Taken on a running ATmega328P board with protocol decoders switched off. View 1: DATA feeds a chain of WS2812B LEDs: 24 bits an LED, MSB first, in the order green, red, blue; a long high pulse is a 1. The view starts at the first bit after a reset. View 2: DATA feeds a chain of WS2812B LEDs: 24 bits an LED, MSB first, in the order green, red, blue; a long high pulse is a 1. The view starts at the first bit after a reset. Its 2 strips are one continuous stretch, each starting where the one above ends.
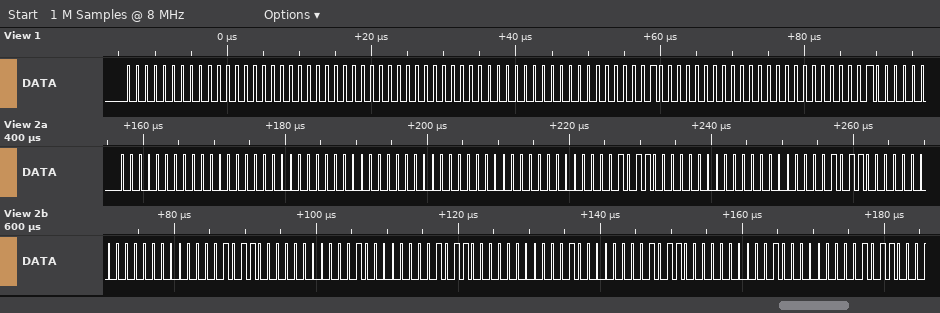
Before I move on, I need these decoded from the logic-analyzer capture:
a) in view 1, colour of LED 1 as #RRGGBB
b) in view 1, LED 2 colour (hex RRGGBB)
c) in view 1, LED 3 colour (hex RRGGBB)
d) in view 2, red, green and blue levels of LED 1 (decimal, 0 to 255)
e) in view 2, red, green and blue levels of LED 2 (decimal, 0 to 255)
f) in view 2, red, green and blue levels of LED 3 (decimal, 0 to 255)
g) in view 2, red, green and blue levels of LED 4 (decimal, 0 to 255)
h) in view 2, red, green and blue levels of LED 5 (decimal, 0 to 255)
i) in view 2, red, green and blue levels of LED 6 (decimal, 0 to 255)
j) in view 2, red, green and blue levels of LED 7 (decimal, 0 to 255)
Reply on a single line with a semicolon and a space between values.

#000000; #000000; #200000; 0, 0, 0; 0, 0, 0; 176, 0, 0; 176, 0, 0; 176, 0, 1; 176, 0, 1; 176, 0, 2
